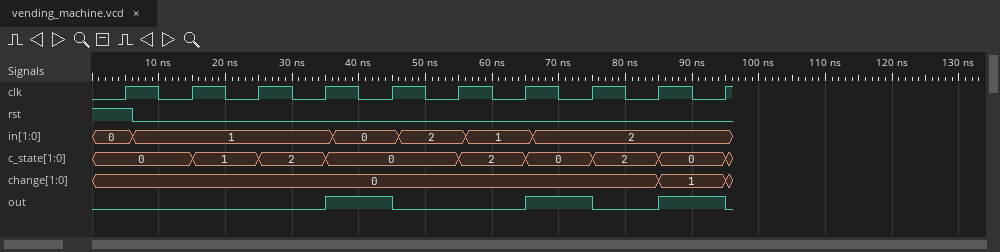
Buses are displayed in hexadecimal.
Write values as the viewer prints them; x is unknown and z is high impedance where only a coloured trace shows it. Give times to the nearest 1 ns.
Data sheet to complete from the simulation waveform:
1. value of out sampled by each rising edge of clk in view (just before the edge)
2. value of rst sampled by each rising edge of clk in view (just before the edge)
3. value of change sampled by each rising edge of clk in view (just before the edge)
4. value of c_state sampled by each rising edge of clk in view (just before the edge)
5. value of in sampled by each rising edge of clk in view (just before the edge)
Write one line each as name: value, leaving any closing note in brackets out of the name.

value of out sampled by each rising edge of clk in view: 0 0 0 0 1 0 0 1 0 1
value of rst sampled by each rising edge of clk in view: 1 0 0 0 0 0 0 0 0 0
value of change sampled by each rising edge of clk in view: 0, 0, 0, 0, 0, 0, 0, 0, 0, 1
value of c_state sampled by each rising edge of clk in view: 0, 0, 1, 2, 0, 0, 2, 0, 2, 0
value of in sampled by each rising edge of clk in view: 0, 1, 1, 1, 0, 2, 1, 2, 2, 2
